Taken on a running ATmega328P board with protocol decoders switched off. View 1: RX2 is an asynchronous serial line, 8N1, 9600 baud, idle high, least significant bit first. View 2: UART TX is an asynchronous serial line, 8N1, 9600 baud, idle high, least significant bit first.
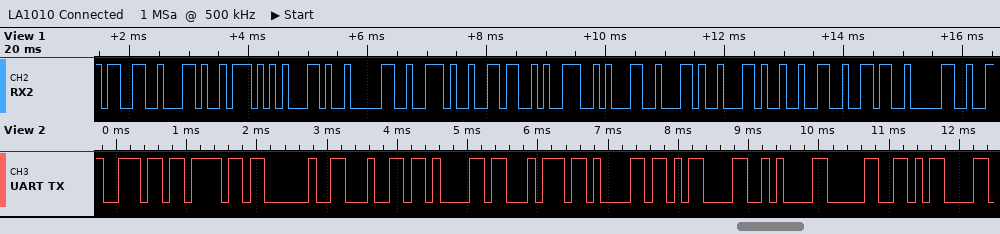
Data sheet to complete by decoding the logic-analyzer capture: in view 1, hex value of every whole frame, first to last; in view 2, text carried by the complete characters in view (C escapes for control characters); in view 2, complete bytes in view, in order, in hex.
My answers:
0x33 0x2C 0x57 0x2C 0x30 0x2E 0x36 0x39 0x31 0x2C 0x2C 0x32 0x36 0x30
"no data\r\n0\r"
0x6E 0x6F 0x20 0x64 0x61 0x74 0x61 0x0D 0x0A 0x30 0x0D
